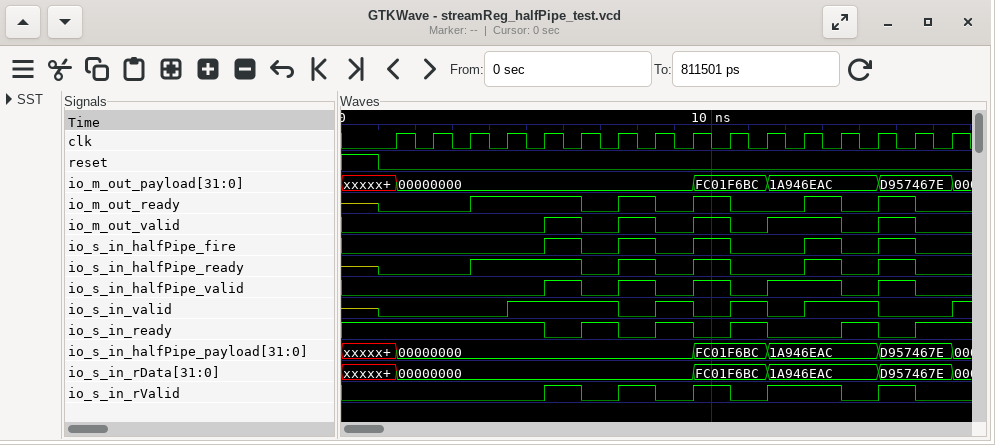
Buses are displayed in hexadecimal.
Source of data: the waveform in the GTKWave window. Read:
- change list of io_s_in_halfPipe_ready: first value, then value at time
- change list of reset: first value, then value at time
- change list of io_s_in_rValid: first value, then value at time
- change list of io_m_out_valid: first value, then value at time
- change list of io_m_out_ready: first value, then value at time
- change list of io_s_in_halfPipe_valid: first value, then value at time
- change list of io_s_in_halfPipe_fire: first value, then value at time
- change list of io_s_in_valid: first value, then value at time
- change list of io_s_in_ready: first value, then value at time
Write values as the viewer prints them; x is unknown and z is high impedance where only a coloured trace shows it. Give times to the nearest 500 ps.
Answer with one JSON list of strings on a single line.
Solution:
["z, 0 at 1000 ps, 1 at 3500 ps, 0 at 6500 ps, 1 at 7500 ps, 0 at 8500 ps, 1 at 9500 ps, 0 at 10500 ps, 1 at 12500 ps, 0 at 13500 ps, 1 at 14500 ps, 0 at 15500 ps", "1, 0 at 1000 ps", "0, 1 at 5500 ps, 0 at 6500 ps, 1 at 7500 ps, 0 at 8500 ps, 1 at 9500 ps, 0 at 10500 ps, 1 at 11500 ps, 0 at 13500 ps, 1 at 14500 ps, 0 at 15500 ps", "0, 1 at 5500 ps, 0 at 6500 ps, 1 at 7500 ps, 0 at 8500 ps, 1 at 9500 ps, 0 at 10500 ps, 1 at 11500 ps, 0 at 13500 ps, 1 at 14500 ps, 0 at 15500 ps", "z, 0 at 1000 ps, 1 at 3500 ps, 0 at 6500 ps, 1 at 7500 ps, 0 at 8500 ps, 1 at 9500 ps, 0 at 10500 ps, 1 at 12500 ps, 0 at 13500 ps, 1 at 14500 ps, 0 at 15500 ps", "0, 1 at 5500 ps, 0 at 6500 ps, 1 at 7500 ps, 0 at 8500 ps, 1 at 9500 ps, 0 at 10500 ps, 1 at 11500 ps, 0 at 13500 ps, 1 at 14500 ps, 0 at 15500 ps", "0, 1 at 5500 ps, 0 at 6500 ps, 1 at 7500 ps, 0 at 8500 ps, 1 at 9500 ps, 0 at 10500 ps, 1 at 12500 ps, 0 at 13500 ps, 1 at 14500 ps, 0 at 15500 ps", "z, 0 at 1000 ps, 1 at 4500 ps, 0 at 7500 ps, 1 at 8500 ps, 0 at 9500 ps, 1 at 10500 ps, 0 at 11500 ps, 1 at 12500 ps, 0 at 14500 ps, 1 at 16500 ps", "1, 0 at 5500 ps, 1 at 6500 ps, 0 at 7500 ps, 1 at 8500 ps, 0 at 9500 ps, 1 at 10500 ps, 0 at 11500 ps, 1 at 13500 ps, 0 at 14500 ps, 1 at 15500 ps"]
